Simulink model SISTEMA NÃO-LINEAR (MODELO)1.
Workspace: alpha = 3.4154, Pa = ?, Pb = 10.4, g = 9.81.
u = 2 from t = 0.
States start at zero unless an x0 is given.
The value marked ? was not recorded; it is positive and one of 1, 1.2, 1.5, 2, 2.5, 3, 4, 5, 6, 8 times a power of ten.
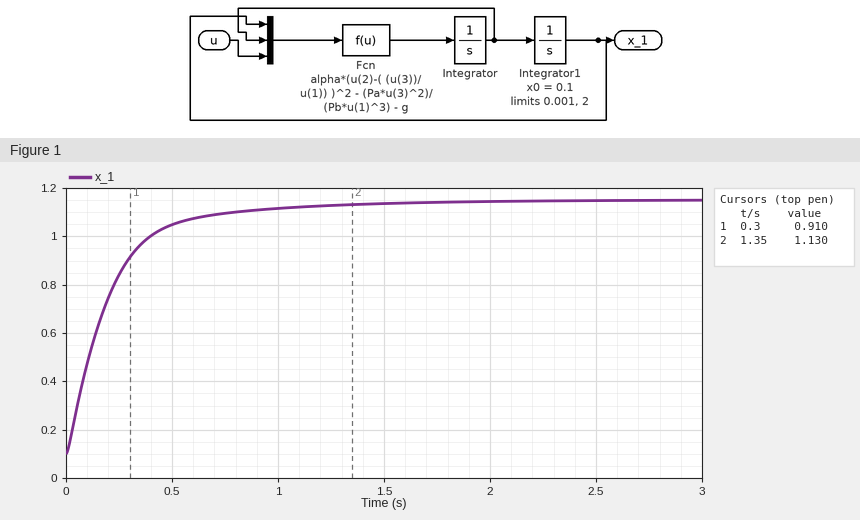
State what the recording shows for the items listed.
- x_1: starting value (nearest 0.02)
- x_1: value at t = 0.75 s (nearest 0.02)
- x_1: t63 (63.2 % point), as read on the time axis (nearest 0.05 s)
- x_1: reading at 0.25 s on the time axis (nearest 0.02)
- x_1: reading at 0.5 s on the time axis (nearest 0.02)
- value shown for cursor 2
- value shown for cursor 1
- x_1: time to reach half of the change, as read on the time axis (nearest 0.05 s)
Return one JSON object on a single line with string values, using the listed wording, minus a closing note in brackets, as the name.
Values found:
{"x_1: starting value": "0.10", "x_1: value at t = 0.75 s": "1.10", "x_1: t63 (63.2 % point), as read on the time axis": "0.20 s", "x_1: reading at 0.25 s on the time axis": "0.84", "x_1: reading at 0.5 s on the time axis": "1.04", "value shown for cursor 2": "1.130", "value shown for cursor 1": "0.910", "x_1: time to reach half of the change, as read on the time axis": "0.15 s"}
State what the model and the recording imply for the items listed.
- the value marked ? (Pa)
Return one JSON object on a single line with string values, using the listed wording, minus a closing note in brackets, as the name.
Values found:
{"the value marked ?": "2"}
